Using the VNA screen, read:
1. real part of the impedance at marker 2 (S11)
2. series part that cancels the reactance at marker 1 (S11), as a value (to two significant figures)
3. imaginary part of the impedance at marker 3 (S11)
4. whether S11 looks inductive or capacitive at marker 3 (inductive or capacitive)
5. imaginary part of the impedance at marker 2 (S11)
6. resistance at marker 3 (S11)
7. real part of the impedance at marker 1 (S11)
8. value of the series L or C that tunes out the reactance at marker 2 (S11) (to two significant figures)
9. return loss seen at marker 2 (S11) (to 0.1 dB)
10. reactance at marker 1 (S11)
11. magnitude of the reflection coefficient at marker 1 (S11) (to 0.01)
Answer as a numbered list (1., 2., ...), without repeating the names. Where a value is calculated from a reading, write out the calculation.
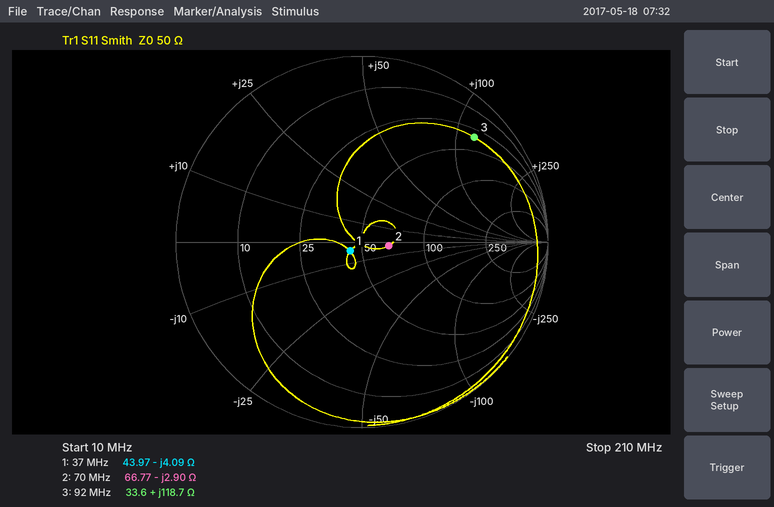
1. 66.77 Ω
2. L = 4.09 Ω/(2π × 37 MHz) ≈ 18 nH
3. +118.7 Ω
4. inductive
5. -2.90 Ω
6. 33.6 Ω
7. 43.97 Ω
8. L = 2.9 Ω/(2π × 70 MHz) ≈ 6.6 nH
9. 16.7 dB
10. -4.09 Ω
11. 0.08
